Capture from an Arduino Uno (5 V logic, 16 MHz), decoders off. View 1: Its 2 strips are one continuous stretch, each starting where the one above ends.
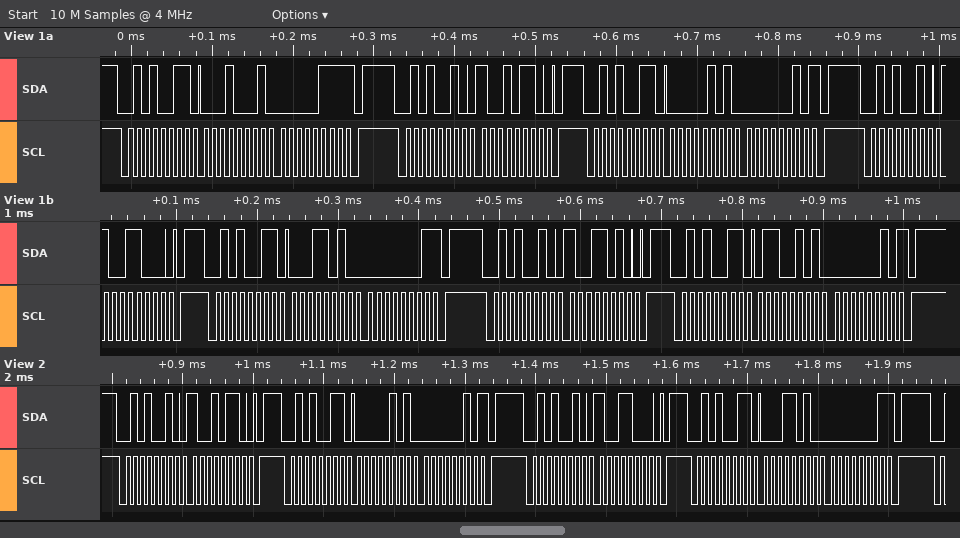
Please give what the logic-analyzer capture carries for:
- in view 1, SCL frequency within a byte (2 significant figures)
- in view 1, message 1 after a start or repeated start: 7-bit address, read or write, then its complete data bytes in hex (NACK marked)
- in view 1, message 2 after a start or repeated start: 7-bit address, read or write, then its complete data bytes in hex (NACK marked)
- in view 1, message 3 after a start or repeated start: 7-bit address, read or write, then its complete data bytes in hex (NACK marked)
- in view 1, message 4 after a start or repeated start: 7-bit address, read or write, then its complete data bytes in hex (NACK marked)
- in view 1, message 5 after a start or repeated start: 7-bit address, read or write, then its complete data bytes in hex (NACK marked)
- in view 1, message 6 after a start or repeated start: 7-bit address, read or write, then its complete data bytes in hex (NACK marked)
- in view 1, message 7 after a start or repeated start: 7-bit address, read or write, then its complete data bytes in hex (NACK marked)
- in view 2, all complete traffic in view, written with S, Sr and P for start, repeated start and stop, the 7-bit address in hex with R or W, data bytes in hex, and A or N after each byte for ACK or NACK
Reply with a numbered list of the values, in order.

1. 100 kHz
2. 0x29 read: 11 07 NACK
3. 0x29 write: 96
4. 0x29 read: 05 02 NACK
5. 0x29 write: 98
6. 0x29 read: 1A 01 NACK
7. 0x29 write: 9A
8. 0x29 read: 65 02 NACK
9. S 29W A 96 A P S 29R A 05 A 02 N P S 29W A 98 A P S 29R A 1A A 01 N P
